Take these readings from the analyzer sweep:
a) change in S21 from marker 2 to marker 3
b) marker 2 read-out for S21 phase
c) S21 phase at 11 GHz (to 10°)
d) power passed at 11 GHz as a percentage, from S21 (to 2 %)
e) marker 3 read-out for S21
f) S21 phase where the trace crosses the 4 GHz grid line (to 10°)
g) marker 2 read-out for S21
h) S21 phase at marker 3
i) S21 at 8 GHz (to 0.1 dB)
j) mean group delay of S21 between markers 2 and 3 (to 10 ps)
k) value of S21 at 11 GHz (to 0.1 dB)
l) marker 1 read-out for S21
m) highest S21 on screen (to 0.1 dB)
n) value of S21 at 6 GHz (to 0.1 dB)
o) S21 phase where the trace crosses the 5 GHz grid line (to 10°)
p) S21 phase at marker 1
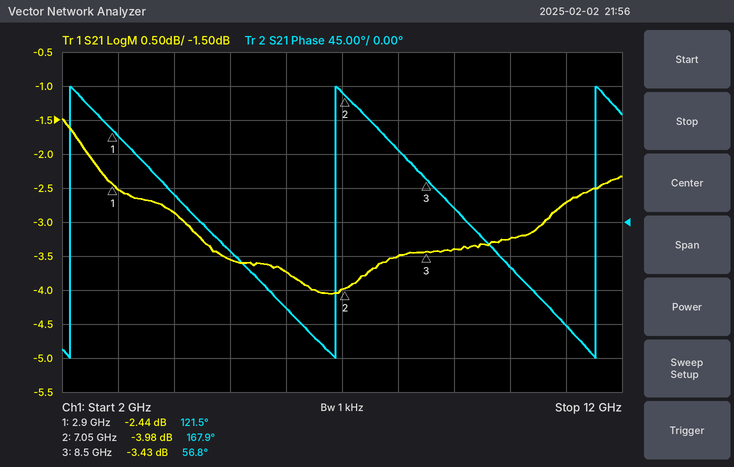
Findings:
0.55 dB
167.9°
-140°
54 %
-3.43 dB
40°
-3.98 dB
56.8°
-3.5 dB
210 ps
-2.7 dB
-2.44 dB
-1.5 dB
-3.7 dB
-40°
121.5°
